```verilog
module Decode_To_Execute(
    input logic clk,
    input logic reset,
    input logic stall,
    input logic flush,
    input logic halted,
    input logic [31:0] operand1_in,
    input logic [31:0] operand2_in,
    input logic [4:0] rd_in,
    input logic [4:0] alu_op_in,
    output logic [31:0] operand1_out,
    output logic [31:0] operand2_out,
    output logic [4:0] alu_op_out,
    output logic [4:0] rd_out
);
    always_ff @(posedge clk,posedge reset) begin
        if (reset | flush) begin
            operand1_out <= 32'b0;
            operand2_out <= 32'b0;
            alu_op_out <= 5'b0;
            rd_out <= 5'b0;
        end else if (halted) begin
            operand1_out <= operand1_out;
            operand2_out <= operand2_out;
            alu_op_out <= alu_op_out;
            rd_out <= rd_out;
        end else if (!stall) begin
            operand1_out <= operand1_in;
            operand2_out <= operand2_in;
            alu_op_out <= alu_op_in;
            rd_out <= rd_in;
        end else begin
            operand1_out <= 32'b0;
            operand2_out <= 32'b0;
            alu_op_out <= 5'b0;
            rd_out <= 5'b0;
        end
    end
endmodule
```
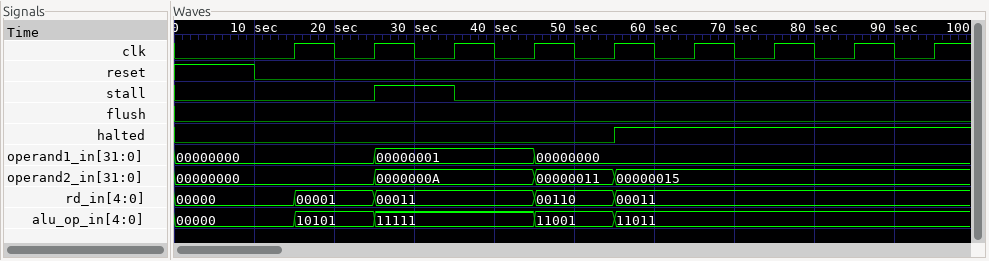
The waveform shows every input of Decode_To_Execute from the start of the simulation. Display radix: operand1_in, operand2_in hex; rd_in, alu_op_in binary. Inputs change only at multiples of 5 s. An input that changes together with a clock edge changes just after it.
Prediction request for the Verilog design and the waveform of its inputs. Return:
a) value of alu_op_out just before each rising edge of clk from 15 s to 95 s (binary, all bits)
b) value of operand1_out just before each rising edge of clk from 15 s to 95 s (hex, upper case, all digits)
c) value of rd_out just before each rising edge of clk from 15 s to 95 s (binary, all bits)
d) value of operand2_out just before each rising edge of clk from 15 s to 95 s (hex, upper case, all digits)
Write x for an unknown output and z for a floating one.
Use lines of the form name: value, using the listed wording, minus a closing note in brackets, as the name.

value of alu_op_out just before each rising edge of clk from 15 s to 95 s: 00000, 00000, 10101, 00000, 11111, 11001, 11001, 11001, 11001
value of operand1_out just before each rising edge of clk from 15 s to 95 s: 00000000, 00000000, 00000000, 00000000, 00000001, 00000000, 00000000, 00000000, 00000000
value of rd_out just before each rising edge of clk from 15 s to 95 s: 00000, 00000, 00001, 00000, 00011, 00110, 00110, 00110, 00110
value of operand2_out just before each rising edge of clk from 15 s to 95 s: 00000000, 00000000, 00000000, 00000000, 0000000A, 00000011, 00000011, 00000011, 00000011
